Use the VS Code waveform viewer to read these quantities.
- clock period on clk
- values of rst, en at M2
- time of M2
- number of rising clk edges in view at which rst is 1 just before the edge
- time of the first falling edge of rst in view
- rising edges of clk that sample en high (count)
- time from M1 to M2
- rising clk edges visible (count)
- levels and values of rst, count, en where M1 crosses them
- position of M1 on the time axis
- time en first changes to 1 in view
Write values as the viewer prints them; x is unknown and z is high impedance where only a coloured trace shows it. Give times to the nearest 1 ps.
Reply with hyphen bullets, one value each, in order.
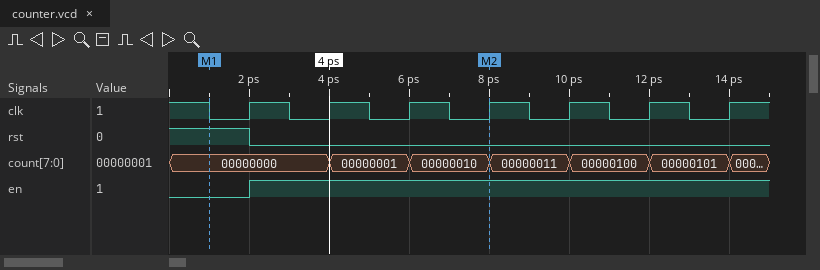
- 2 ps
- rst=0, en=1
- 8 ps
- 1
- 2 ps
- 6
- 7 ps
- 7
- rst=1, count=00000000, en=0
- 1 ps
- 2 ps
